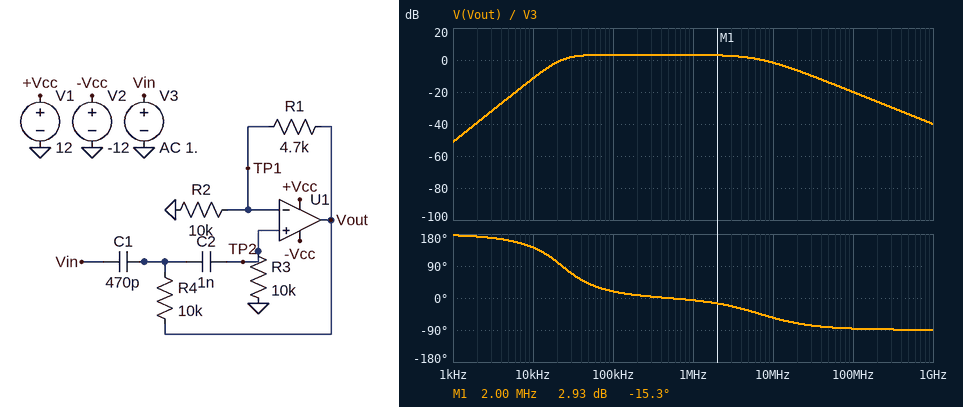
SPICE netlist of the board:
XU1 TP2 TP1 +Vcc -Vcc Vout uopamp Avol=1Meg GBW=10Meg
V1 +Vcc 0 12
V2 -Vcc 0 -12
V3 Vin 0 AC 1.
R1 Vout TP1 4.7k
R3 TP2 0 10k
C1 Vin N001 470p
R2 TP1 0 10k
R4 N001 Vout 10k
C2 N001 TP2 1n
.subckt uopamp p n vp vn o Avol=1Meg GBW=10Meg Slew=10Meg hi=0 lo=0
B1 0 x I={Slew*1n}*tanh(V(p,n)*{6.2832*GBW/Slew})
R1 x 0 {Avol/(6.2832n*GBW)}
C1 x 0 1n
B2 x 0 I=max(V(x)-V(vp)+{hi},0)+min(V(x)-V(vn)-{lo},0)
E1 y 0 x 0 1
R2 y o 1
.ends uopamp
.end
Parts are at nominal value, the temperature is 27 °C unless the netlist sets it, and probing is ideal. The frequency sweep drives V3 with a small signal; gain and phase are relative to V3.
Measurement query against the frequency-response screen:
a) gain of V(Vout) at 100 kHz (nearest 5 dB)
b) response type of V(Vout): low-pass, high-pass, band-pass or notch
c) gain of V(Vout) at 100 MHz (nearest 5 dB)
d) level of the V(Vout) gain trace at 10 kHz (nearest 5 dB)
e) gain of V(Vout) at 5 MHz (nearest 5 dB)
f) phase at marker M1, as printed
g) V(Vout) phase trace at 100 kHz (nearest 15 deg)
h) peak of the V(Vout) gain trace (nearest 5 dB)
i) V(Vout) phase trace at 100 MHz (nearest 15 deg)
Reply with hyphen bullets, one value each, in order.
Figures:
- 5 dB
- band-pass
- -20 dB
- -10 dB
- 0 dB
- -15.3 deg
- 15 deg
- 5 dB
- -90 deg
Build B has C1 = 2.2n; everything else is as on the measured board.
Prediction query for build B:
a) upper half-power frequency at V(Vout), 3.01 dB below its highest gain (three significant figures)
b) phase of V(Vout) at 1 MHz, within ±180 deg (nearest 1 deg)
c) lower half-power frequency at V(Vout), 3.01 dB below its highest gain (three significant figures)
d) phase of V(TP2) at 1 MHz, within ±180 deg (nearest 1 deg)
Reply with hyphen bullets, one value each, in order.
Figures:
- 6.84 MHz
- -7 deg
- 14.8 kHz
- 1 deg
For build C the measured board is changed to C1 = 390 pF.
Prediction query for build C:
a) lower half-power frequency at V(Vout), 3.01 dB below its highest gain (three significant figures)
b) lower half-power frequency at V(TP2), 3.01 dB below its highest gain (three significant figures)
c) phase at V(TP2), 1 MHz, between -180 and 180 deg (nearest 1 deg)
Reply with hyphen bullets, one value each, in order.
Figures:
- 26.3 kHz
- 26.6 kHz
- 2 deg
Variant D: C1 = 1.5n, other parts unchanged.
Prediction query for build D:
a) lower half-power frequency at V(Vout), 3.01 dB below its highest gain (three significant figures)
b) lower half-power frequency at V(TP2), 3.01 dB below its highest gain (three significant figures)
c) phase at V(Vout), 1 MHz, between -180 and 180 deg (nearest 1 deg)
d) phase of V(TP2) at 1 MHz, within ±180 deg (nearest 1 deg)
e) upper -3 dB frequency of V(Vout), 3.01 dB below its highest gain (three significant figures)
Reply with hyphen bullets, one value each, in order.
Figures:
- 15.5 kHz
- 15.6 kHz
- -7 deg
- 1 deg
- 6.84 MHz
